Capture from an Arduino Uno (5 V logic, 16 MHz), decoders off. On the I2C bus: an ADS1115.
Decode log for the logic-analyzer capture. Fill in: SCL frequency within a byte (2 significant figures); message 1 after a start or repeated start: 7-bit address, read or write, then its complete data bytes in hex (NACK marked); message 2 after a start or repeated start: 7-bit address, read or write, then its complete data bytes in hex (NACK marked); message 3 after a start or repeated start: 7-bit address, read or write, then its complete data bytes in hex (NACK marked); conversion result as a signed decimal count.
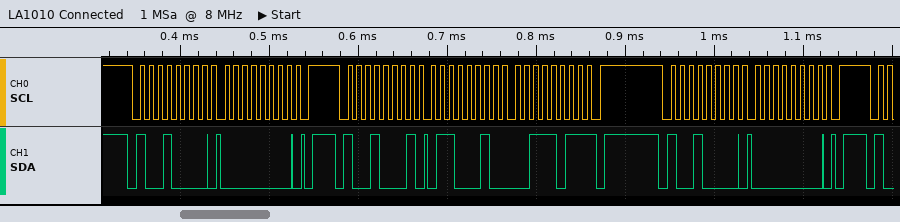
100 kHz
0x48 write: 00
0x48 read: 62 3B NACK
0x48 write: 00
25147
